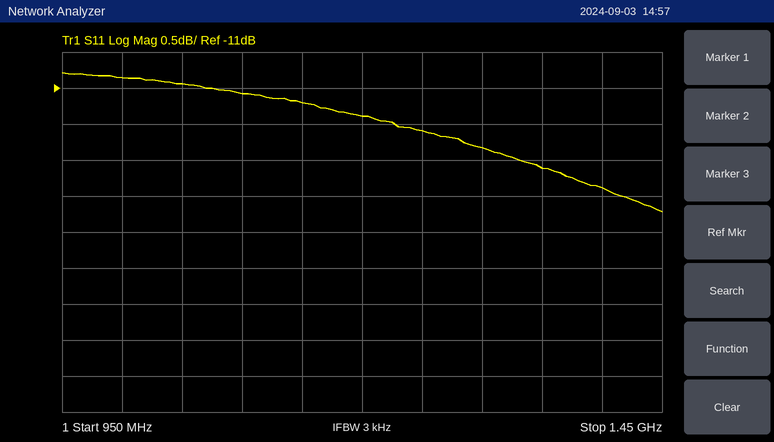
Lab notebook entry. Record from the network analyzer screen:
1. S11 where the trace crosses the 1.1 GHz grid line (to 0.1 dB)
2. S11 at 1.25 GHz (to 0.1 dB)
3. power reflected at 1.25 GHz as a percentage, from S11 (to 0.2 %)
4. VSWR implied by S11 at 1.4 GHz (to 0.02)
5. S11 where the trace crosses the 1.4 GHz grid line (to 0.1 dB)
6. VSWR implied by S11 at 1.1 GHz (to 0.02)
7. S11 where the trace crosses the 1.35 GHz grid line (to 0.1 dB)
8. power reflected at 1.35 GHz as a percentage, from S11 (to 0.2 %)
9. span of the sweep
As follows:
-11.1 dB
-11.6 dB
7.0 %
1.64
-12.4 dB
1.78
-12.1 dB
6.2 %
500 MHz
